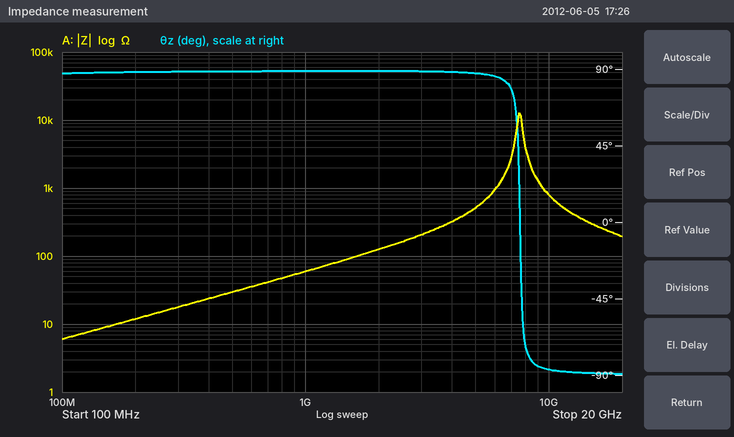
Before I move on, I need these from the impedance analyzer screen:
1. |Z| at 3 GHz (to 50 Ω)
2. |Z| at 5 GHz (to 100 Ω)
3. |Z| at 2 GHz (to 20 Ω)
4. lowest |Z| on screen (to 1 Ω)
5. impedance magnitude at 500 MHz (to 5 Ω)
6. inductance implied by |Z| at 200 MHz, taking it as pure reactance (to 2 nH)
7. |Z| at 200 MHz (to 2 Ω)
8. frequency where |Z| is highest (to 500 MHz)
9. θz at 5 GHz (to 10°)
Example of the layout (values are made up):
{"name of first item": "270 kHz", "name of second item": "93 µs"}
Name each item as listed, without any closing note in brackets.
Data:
{"|Z| at 3 GHz": "200 Ω", "|Z| at 5 GHz": "500 Ω", "|Z| at 2 GHz": "120 Ω", "lowest |Z| on screen": "6 Ω", "impedance magnitude at 500 MHz": "30 Ω", "inductance implied by |Z| at 200 MHz, taking it as pure reactance": "10 nH", "|Z| at 200 MHz": "12 Ω", "frequency where |Z| is highest": "7.5 GHz", "θz at 5 GHz": "90°"}
